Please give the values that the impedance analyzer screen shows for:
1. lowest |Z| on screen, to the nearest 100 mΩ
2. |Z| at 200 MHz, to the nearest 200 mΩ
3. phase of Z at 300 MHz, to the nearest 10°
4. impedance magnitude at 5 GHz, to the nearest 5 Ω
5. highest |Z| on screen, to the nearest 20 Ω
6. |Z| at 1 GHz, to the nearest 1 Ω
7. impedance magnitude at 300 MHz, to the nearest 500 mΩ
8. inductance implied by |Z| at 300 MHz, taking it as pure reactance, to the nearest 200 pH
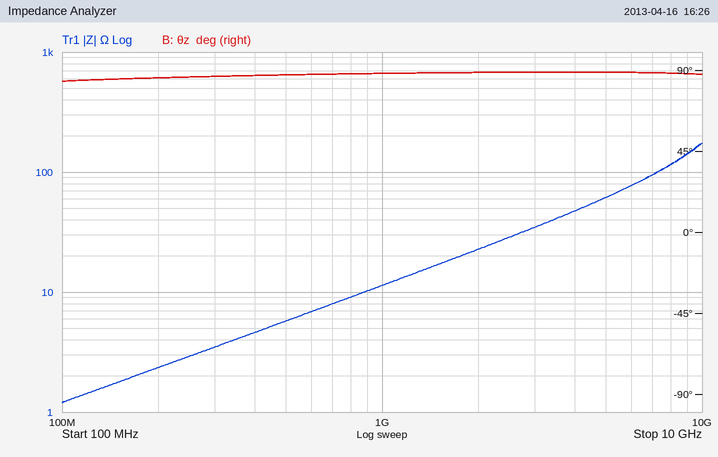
1.2 Ω
2.4 Ω
90°
60 Ω
180 Ω
11 Ω
3.5 Ω
1.8 nH
